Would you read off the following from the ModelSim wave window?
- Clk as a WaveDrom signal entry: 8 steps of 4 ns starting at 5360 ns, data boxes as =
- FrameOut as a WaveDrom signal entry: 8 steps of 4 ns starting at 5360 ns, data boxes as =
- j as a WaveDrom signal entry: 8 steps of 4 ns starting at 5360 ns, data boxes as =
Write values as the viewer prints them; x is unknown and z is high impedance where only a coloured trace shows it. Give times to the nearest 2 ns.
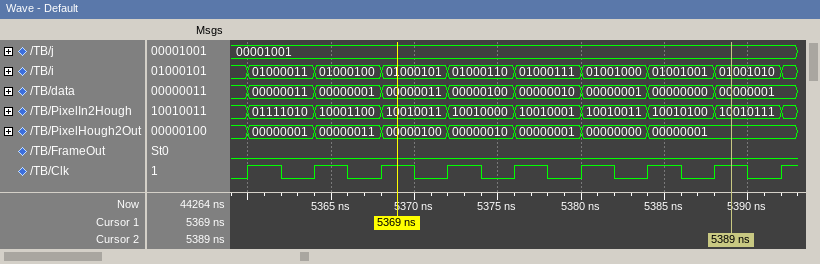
{name: 'Clk', wave: 'p.......'}
{name: 'FrameOut', wave: '0.......'}
{name: 'j', wave: '=.......', data: '00001001'}
